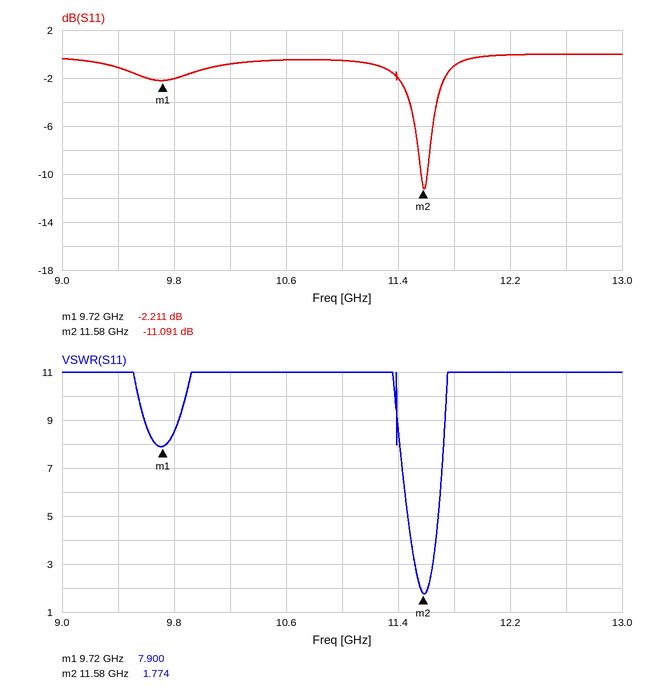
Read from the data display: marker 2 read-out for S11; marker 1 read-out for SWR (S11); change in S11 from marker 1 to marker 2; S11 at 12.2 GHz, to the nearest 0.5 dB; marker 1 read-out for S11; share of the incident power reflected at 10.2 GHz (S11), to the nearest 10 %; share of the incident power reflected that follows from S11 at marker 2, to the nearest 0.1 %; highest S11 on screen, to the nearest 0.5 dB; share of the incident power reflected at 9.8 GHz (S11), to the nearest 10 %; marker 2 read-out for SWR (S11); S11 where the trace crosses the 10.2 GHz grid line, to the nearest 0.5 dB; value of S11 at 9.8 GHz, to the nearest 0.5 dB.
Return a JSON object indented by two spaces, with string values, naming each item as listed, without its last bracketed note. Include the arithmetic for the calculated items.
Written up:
{
  "marker 2 read-out for S11": "-11.091 dB",
  "marker 1 read-out for SWR": "7.900",
  "change in S11 from marker 1 to marker 2": "-11.091 − (-2.211) = -8.880 dB",
  "S11 at 12.2 GHz, to the nearest 0.5 dB": "0.0 dB",
  "marker 1 read-out for S11": "-2.211 dB",
  "share of the incident power reflected at 10.2 GHz (S11), to the nearest 10 %": "10^(-1/10) ≈ 79.4 %, so 80 % to the nearest 10 %",
  "share of the incident power reflected that follows from S11 at marker 2, to the nearest 0.1 %": "10^(-11.091/10) ≈ 7.8 %",
  "highest S11 on screen, to the nearest 0.5 dB": "0.0 dB",
  "share of the incident power reflected at 9.8 GHz (S11), to the nearest 10 %": "10^(-2/10) ≈ 63.1 %, so 60 % to the nearest 10 %",
  "marker 2 read-out for SWR": "1.774",
  "S11 where the trace crosses the 10.2 GHz grid line, to the nearest 0.5 dB": "-1.0 dB",
  "value of S11 at 9.8 GHz, to the nearest 0.5 dB": "-2.0 dB"
}
